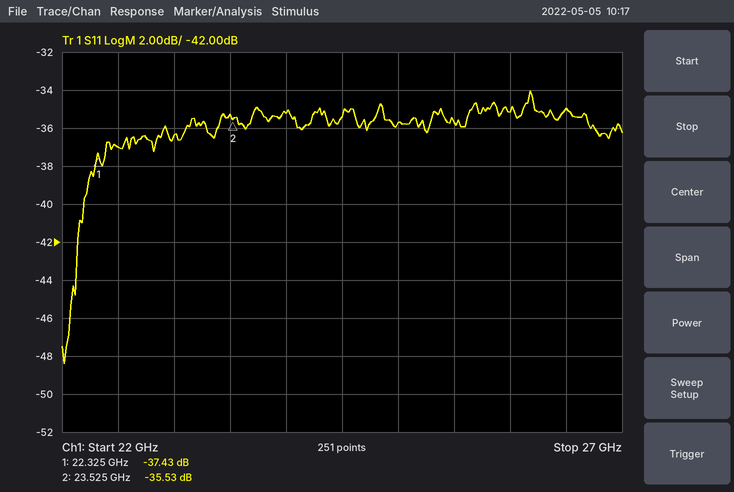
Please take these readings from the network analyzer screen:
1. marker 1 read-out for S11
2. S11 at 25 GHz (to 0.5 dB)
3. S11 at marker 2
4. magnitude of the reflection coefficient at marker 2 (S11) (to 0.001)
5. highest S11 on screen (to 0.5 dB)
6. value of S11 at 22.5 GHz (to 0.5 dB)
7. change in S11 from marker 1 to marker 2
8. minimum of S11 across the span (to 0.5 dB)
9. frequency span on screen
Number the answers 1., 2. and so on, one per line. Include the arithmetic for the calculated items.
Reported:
1. -37.43 dB
2. -35.5 dB
3. -35.53 dB
4. 10^(-35.53/20) ≈ 0.017
5. -34.0 dB
6. -37.0 dB
7. -35.53 − (-37.43) = 1.90 dB
8. -48.5 dB
9. 5 GHz
